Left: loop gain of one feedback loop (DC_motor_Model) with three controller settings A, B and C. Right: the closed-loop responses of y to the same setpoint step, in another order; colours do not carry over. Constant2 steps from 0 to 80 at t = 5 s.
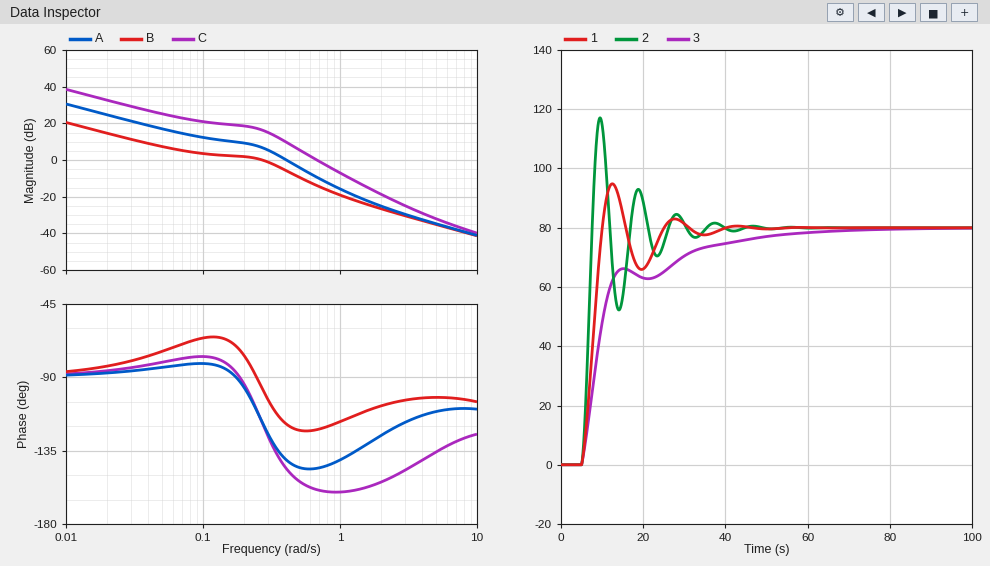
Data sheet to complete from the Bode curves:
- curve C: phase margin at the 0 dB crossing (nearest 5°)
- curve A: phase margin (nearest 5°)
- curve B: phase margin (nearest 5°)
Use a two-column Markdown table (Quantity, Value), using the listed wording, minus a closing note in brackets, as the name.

| Quantity | Value |
|---|---|
| curve C: phase margin at the 0 dB crossing | 20° |
| curve A: phase margin | 40° |
| curve B: phase margin | 85° |
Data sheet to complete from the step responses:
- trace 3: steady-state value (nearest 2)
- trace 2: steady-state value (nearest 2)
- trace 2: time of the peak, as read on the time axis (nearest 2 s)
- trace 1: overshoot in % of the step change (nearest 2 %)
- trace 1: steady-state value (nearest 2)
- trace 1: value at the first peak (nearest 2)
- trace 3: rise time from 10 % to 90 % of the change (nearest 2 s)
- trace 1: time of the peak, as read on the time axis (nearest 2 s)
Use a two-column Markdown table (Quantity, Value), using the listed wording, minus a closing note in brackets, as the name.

| Quantity | Value |
|---|---|
| trace 3: steady-state value | 80 |
| trace 2: steady-state value | 80 |
| trace 2: time of the peak, as read on the time axis | 10 s |
| trace 1: overshoot in % of the step change | 18 % |
| trace 1: steady-state value | 80 |
| trace 1: value at the first peak | 94 |
| trace 3: rise time from 10 % to 90 % of the change | 26 s |
| trace 1: time of the peak, as read on the time axis | 12 s |
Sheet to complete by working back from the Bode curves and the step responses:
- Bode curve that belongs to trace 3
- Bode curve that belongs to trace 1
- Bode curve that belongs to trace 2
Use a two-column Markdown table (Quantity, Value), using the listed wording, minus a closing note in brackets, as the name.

| Quantity | Value |
|---|---|
| Bode curve that belongs to trace 3 | B |
| Bode curve that belongs to trace 1 | A |
| Bode curve that belongs to trace 2 | C |
